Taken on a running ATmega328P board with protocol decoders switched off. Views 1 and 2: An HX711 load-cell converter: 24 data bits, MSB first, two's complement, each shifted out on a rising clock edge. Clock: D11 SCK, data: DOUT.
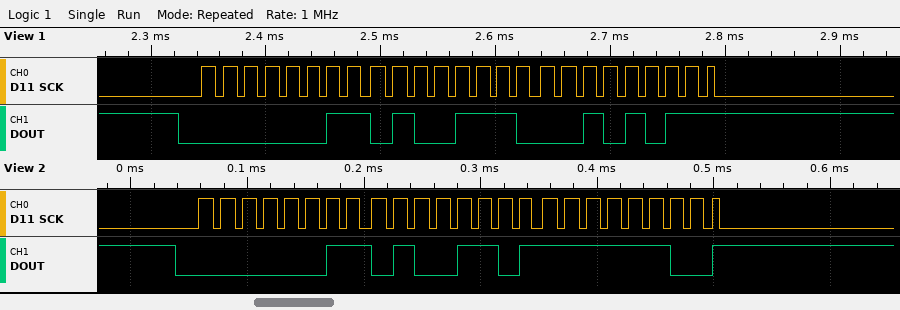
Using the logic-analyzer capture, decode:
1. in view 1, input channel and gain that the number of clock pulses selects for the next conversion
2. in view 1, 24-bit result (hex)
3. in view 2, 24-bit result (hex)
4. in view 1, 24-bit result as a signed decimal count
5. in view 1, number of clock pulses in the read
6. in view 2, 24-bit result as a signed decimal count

channel A, gain 128
0x034E2B
0x034DFC
216619
25
216572
